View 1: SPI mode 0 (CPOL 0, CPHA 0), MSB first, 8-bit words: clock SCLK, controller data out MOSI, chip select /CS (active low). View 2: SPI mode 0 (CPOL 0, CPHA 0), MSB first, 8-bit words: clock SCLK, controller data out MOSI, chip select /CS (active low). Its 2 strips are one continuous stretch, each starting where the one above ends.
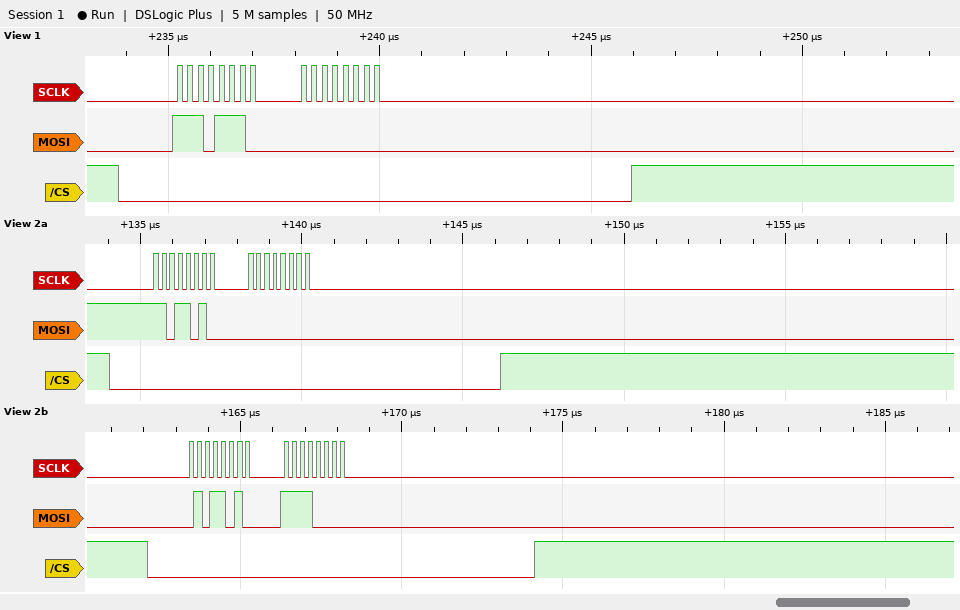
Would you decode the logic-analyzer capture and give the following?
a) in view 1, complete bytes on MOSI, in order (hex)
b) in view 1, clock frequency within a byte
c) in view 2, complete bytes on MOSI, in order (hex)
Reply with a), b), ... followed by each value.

a) 0xEE 0x00
b) 4 MHz
c) DA 00 5A F0
